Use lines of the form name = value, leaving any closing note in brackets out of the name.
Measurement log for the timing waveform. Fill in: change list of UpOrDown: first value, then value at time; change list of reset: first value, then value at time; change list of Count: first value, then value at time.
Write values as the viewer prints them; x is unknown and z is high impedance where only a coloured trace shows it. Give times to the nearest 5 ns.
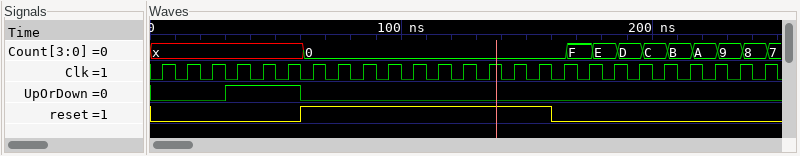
change list of UpOrDown: first value, then value at time = 0, 1 at 30 ns, 0 at 60 ns
change list of reset: first value, then value at time = 0, 1 at 60 ns, 0 at 160 ns
change list of Count: first value, then value at time = x, 0 at 60 ns, F at 165 ns, E at 175 ns, D at 185 ns, C at 195 ns, B at 205 ns, A at 215 ns, 9 at 225 ns, 8 at 235 ns, 7 at 245 ns
